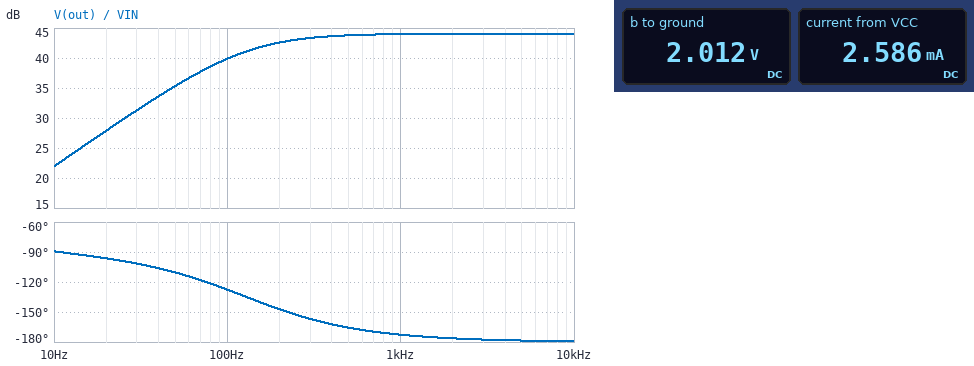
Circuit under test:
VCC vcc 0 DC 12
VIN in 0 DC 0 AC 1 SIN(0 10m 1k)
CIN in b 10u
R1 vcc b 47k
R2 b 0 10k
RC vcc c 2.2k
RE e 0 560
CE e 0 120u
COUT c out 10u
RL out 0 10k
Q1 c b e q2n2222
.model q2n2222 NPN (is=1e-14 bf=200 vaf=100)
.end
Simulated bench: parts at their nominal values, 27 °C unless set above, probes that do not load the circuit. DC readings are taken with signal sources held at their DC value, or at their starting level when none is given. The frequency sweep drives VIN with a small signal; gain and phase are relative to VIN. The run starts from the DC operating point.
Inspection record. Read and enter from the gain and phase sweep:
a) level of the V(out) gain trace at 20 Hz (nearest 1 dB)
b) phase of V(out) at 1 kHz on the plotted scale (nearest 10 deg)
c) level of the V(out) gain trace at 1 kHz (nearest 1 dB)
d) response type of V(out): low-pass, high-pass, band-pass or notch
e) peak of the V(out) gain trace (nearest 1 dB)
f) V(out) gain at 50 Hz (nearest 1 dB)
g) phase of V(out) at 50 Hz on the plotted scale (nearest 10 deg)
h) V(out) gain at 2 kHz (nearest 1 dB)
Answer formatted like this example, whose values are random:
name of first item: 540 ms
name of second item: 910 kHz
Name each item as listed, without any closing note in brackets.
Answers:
level of the V(out) gain trace at 20 Hz: 28 dB
phase of V(out) at 1 kHz on the plotted scale: -170 deg
level of the V(out) gain trace at 1 kHz: 44 dB
response type of V(out): low-pass, high-pass, band-pass or notch: high-pass
peak of the V(out) gain trace: 44 dB
V(out) gain at 50 Hz: 35 dB
phase of V(out) at 50 Hz on the plotted scale: -110 deg
V(out) gain at 2 kHz: 44 dB
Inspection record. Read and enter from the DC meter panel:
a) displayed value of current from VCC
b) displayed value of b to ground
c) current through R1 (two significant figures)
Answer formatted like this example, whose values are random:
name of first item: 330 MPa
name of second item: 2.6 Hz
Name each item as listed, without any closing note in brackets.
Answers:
displayed value of current from VCC: 2.586 mA
displayed value of b to ground: 2.012 V
current through R1: 210 µA
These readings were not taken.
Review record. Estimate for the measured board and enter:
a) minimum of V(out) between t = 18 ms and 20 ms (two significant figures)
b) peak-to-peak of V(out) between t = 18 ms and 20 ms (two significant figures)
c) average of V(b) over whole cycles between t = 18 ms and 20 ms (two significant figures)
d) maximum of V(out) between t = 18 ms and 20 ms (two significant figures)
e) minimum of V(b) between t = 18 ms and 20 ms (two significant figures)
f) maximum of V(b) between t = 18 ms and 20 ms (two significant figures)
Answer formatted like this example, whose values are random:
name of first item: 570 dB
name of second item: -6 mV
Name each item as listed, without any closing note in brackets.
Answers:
minimum of V(out) between t = 18 ms and 20 ms: -1.7 V
peak-to-peak of V(out) between t = 18 ms and 20 ms: 3.1 V
average of V(b) over whole cycles between t = 18 ms and 20 ms: 2.0 V
maximum of V(out) between t = 18 ms and 20 ms: 1.4 V
minimum of V(b) between t = 18 ms and 20 ms: 2.0 V
maximum of V(b) between t = 18 ms and 20 ms: 2.0 V
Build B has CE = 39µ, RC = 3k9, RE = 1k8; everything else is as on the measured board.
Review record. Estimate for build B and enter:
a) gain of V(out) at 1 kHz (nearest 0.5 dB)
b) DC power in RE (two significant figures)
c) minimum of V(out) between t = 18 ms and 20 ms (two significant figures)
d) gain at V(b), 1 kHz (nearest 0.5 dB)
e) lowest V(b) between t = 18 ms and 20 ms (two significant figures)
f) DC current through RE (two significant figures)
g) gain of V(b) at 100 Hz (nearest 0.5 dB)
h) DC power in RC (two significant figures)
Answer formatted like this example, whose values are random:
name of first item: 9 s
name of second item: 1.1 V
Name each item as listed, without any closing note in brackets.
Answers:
gain of V(out) at 1 kHz: 38.5 dB
DC power in RE: 1.1 mW
minimum of V(out) between t = 18 ms and 20 ms: -900 mV
gain at V(b), 1 kHz: 0 dB
lowest V(b) between t = 18 ms and 20 ms: 2.1 V
DC current through RE: 790 µA
gain of V(b) at 100 Hz: 0 dB
DC power in RC: 2.4 mW
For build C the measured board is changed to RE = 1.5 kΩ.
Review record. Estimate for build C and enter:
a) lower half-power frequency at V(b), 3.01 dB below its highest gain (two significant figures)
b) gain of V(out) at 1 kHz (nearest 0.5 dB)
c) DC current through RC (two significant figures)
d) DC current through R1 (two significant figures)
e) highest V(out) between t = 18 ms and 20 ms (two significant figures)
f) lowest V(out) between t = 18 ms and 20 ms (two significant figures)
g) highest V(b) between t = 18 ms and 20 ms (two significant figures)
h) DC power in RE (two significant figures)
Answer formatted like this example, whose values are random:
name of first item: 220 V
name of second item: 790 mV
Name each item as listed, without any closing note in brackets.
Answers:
lower half-power frequency at V(b), 3.01 dB below its highest gain: 2.1 Hz
gain of V(out) at 1 kHz: 36.0 dB
DC current through RC: 940 µA
DC current through R1: 210 µA
highest V(out) between t = 18 ms and 20 ms: 580 mV
lowest V(out) between t = 18 ms and 20 ms: -700 mV
highest V(b) between t = 18 ms and 20 ms: 2.1 V
DC power in RE: 1.3 mW
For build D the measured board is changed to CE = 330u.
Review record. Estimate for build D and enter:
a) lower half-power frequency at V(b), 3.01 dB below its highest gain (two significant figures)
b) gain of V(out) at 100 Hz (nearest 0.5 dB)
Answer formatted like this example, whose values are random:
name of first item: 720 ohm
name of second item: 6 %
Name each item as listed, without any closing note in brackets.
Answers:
lower half-power frequency at V(b), 3.01 dB below its highest gain: 2.6 Hz
gain of V(out) at 100 Hz: 43.0 dB
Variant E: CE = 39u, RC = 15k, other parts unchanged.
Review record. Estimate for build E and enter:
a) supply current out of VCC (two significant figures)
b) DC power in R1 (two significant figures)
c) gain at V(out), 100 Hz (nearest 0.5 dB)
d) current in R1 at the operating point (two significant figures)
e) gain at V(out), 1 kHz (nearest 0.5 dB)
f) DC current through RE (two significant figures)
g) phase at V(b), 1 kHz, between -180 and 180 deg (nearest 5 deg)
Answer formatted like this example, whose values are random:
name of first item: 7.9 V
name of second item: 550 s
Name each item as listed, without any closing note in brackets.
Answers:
supply current out of VCC: 990 µA
DC power in R1: 2.5 mW
gain at V(out), 100 Hz: -1.5 dB
current in R1 at the operating point: 230 µA
gain at V(out), 1 kHz: 10.0 dB
DC current through RE: 880 µA
phase at V(b), 1 kHz, between -180 and 180 deg: 15 deg
